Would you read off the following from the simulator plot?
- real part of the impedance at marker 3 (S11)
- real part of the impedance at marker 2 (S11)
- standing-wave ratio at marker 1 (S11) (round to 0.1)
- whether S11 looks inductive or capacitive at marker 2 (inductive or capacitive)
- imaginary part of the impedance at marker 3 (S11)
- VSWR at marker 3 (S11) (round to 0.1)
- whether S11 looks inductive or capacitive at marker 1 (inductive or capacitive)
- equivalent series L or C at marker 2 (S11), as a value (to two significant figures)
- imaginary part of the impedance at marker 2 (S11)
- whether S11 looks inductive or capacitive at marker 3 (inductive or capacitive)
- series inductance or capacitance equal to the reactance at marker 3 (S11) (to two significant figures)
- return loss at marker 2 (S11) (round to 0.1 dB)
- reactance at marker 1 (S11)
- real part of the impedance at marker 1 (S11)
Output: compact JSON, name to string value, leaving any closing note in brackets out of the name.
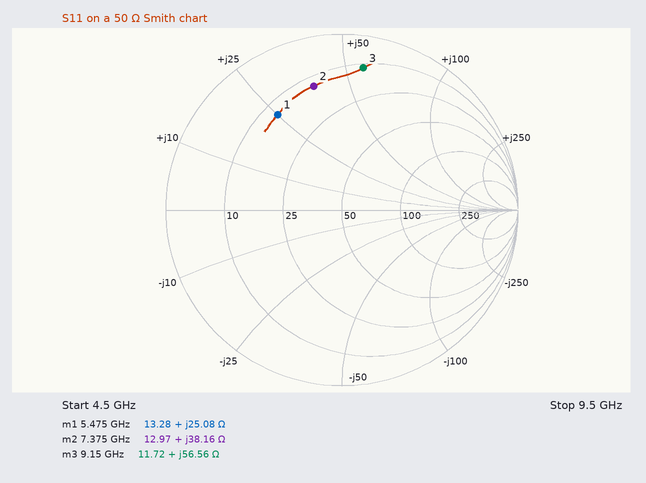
{"real part of the impedance at marker 3": "11.72 Ω", "real part of the impedance at marker 2": "12.97 Ω", "standing-wave ratio at marker 1 (S11)": "4.8", "whether S11 looks inductive or capacitive at marker 2": "inductive", "imaginary part of the impedance at marker 3": "+56.56 Ω", "VSWR at marker 3 (S11)": "9.9", "whether S11 looks inductive or capacitive at marker 1": "inductive", "equivalent series L or C at marker 2 (S11), as a value": "820 pH", "imaginary part of the impedance at marker 2": "+38.16 Ω", "whether S11 looks inductive or capacitive at marker 3": "inductive", "series inductance or capacitance equal to the reactance at marker 3 (S11)": "980 pH", "return loss at marker 2 (S11)": "2.8 dB", "reactance at marker 1": "+25.08 Ω", "real part of the impedance at marker 1": "13.28 Ω"}
